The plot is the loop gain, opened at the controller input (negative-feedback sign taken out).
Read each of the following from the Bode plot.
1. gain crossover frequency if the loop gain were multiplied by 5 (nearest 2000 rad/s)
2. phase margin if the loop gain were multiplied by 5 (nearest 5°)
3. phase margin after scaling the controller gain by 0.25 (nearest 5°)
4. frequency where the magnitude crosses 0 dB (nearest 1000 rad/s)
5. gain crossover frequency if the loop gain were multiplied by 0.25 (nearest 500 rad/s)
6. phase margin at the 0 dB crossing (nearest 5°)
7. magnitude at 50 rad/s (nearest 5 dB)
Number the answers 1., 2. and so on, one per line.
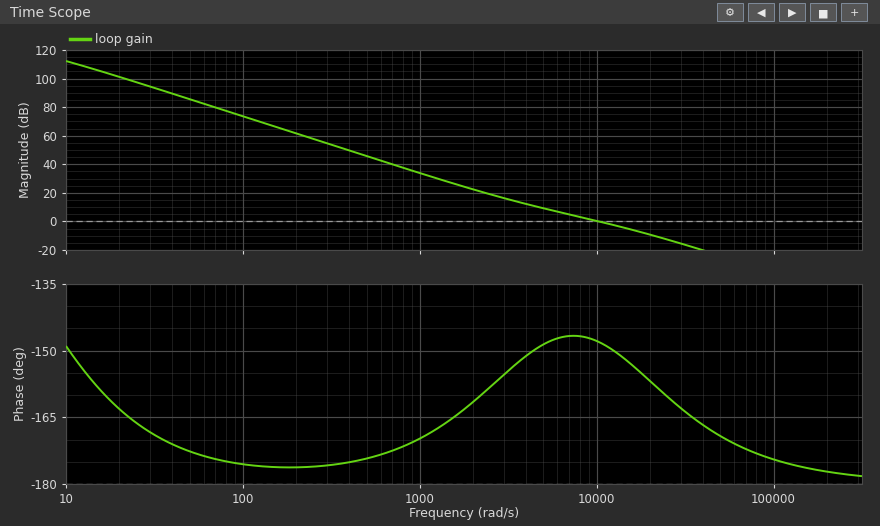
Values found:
1. 28000 rad/s
2. 20°
3. 30°
4. 10000 rad/s
5. 4000 rad/s
6. 30°
7. 85 dB
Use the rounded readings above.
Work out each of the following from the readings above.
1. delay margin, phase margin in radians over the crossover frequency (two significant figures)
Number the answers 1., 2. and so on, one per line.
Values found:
1. 0.000052 s
